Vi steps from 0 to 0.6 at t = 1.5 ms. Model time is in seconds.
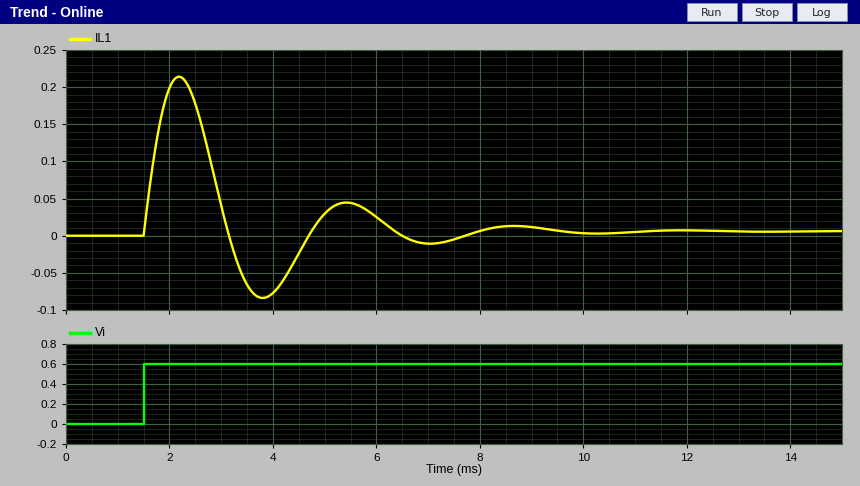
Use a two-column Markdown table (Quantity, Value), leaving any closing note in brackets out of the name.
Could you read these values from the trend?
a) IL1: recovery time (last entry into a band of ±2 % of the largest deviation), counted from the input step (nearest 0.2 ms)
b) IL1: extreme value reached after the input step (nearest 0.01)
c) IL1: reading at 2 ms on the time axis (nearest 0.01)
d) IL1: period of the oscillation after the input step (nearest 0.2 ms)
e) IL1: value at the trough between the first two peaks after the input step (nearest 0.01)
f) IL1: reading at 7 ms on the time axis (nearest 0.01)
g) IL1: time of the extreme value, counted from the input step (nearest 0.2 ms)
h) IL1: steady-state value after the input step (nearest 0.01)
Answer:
| Quantity | Value |
|---|---|
| IL1: recovery time (last entry into a band of ±2 % of the largest deviation), counted from the input step | 7.6 ms |
| IL1: extreme value reached after the input step | 0.21 |
| IL1: reading at 2 ms on the time axis | 0.20 |
| IL1: period of the oscillation after the input step | 3.2 ms |
| IL1: value at the trough between the first two peaks after the input step | -0.08 |
| IL1: reading at 7 ms on the time axis | -0.01 |
| IL1: time of the extreme value, counted from the input step | 0.6 ms |
| IL1: steady-state value after the input step | 0.01 |
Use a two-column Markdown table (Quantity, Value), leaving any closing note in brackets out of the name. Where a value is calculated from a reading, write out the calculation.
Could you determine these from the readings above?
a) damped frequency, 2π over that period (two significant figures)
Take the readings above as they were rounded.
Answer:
| Quantity | Value |
|---|---|
| damped frequency, 2π over that period | 2π / 3.2 = 2.0 rad/ms |
